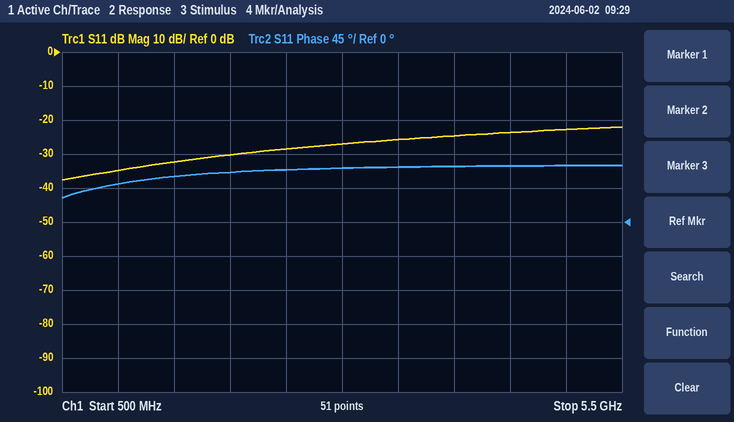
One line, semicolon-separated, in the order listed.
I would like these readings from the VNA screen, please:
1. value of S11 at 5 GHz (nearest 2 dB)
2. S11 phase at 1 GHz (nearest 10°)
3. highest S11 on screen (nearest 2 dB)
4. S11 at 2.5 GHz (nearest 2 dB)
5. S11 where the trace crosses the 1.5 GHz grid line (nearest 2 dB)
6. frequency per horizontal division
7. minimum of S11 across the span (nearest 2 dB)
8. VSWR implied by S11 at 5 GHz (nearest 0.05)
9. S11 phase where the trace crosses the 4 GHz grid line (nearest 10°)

-22 dB; 50°; -22 dB; -28 dB; -32 dB; 500 MHz; -38 dB; 1.15; 70°
